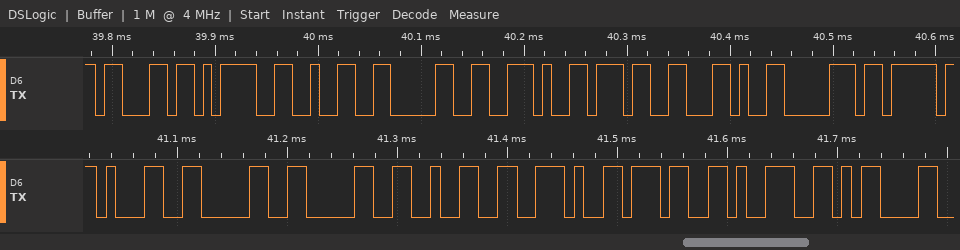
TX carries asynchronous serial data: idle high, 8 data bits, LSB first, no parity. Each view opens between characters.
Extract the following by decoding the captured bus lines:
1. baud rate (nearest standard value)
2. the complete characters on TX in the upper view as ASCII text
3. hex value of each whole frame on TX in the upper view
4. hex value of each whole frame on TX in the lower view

115200 baud
"c=20.7,p"
63, 3D, 32, 30, 2E, 37, 2C, 70
31, 30, 30, 32, 2E, 37, 39, 0D
